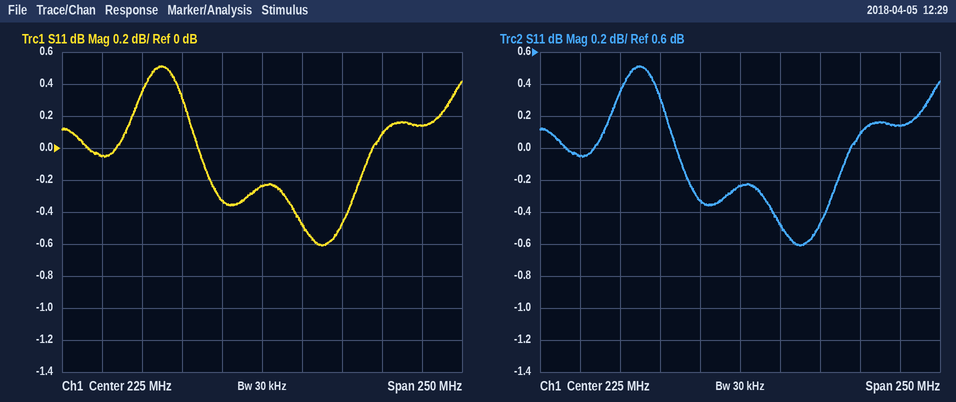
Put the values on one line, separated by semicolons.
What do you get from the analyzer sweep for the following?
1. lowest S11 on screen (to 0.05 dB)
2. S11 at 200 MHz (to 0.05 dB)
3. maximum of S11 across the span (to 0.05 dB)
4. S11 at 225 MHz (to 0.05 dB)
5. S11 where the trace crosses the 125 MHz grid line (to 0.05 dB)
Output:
-0.60 dB; -0.35 dB; 0.50 dB; -0.25 dB; -0.05 dB
